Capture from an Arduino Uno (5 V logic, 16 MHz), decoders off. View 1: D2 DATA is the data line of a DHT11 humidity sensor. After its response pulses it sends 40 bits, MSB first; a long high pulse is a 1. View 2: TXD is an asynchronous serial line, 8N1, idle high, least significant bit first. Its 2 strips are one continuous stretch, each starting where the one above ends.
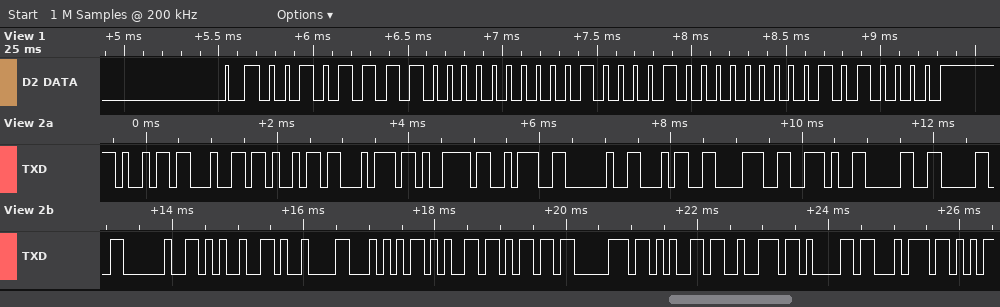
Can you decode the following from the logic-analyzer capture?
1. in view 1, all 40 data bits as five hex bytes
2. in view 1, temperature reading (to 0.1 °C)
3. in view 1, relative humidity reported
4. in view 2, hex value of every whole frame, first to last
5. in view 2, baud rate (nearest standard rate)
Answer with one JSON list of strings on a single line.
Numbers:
["2F 00 21 00 50", "33.0 °C", "47 %", "69 64 69 74 79 3A 20 34 38 2E 30 30 20 25 09 54 65 6D 70 65 72 61 74", "9600 baud"]
